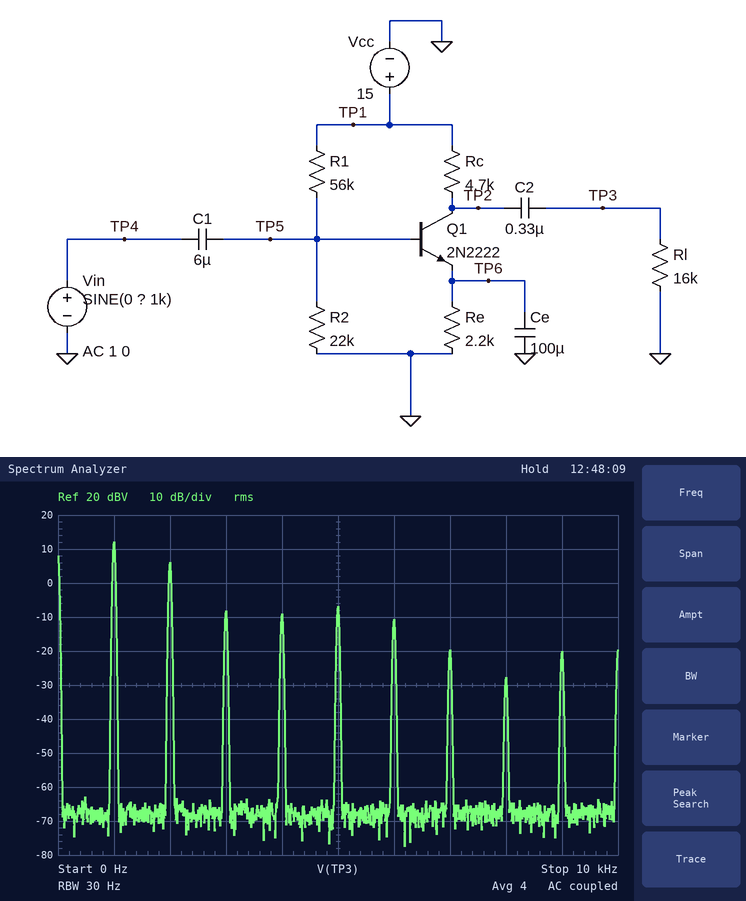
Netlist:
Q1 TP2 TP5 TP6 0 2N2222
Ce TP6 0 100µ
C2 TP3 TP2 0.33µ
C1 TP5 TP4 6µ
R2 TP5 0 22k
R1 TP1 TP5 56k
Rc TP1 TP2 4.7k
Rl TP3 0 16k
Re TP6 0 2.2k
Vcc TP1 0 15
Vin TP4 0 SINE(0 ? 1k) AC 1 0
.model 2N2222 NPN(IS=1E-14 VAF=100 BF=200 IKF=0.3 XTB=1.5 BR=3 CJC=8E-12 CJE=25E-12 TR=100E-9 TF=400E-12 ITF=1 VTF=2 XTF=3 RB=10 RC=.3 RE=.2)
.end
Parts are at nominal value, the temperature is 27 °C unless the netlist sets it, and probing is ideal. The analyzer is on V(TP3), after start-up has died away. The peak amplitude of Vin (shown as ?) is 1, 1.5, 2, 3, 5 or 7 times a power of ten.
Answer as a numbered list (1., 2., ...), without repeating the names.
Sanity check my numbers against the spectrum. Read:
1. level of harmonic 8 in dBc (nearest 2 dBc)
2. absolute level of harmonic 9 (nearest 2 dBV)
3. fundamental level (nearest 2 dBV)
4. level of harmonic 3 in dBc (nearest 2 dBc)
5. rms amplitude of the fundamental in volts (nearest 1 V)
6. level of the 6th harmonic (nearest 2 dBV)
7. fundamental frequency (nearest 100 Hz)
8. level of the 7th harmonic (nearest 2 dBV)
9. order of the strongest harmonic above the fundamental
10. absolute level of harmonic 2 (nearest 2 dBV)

1. -40 dBc
2. -20 dBV
3. 12 dBV
4. -20 dBc
5. 4 V
6. -10 dBV
7. 1.0 kHz
8. -20 dBV
9. 2
10. 6 dBV
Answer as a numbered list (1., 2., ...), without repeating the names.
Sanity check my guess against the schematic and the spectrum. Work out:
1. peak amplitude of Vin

1. 100 mV
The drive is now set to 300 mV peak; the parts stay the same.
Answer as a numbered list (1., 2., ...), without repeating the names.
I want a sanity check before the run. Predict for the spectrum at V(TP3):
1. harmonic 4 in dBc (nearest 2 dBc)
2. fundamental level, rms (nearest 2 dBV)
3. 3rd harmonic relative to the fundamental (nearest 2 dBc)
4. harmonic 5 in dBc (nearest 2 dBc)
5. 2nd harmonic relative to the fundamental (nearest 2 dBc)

1. -14 dBc
2. 10 dBV
3. -6 dBc
4. -40 dBc
5. -2 dBc
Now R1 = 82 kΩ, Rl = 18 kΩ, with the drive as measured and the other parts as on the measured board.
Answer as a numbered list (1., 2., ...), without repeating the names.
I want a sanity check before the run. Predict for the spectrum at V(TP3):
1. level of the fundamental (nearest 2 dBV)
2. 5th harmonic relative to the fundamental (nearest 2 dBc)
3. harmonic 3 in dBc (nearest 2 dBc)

1. 12 dBV
2. -24 dBc
3. -14 dBc
